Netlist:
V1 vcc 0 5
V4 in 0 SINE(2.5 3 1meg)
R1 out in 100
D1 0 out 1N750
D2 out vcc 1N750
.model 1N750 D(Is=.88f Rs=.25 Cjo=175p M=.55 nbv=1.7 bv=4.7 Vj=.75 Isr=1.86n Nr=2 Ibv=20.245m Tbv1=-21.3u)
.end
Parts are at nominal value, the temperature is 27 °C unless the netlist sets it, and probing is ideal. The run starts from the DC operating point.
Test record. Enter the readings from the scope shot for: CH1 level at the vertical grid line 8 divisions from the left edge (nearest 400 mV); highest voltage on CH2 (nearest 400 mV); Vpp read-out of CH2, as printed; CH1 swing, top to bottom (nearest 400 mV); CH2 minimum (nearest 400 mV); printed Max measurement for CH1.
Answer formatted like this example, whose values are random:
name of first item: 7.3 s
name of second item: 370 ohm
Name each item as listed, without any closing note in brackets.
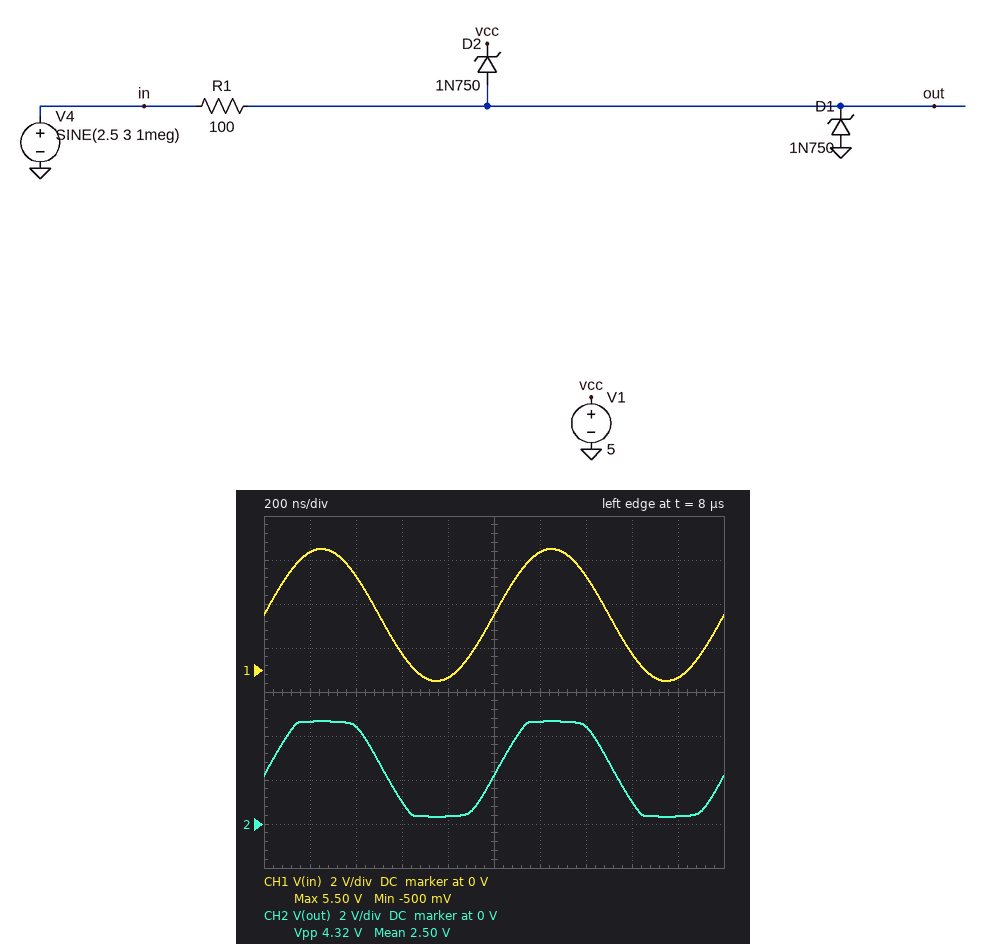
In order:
CH1 level at the vertical grid line 8 divisions from the left edge: 800 mV
highest voltage on CH2: 4.8 V
Vpp read-out of CH2, as printed: 4.32 V
CH1 swing, top to bottom: 6.0 V
CH2 minimum: 400 mV
printed Max measurement for CH1: 5.50 V
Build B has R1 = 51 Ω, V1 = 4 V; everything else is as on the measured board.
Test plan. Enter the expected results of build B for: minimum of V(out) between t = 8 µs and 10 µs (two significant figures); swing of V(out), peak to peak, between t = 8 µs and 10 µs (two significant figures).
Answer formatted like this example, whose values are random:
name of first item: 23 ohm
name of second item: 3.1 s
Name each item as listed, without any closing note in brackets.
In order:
minimum of V(out) between t = 8 µs and 10 µs: -480 mV
swing of V(out), peak to peak, between t = 8 µs and 10 µs: 5.2 V
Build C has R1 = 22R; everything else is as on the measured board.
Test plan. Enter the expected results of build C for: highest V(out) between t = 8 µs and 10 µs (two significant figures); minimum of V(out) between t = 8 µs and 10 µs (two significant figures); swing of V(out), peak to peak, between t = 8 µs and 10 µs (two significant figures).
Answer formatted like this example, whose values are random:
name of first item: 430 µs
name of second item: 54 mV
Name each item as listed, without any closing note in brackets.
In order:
highest V(out) between t = 8 µs and 10 µs: 4.7 V
minimum of V(out) between t = 8 µs and 10 µs: 270 mV
swing of V(out), peak to peak, between t = 8 µs and 10 µs: 4.5 V
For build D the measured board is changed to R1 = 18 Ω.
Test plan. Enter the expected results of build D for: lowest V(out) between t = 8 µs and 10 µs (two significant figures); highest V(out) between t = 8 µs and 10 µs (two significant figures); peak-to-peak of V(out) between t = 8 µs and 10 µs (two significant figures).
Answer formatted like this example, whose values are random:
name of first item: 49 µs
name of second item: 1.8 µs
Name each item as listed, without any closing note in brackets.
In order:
lowest V(out) between t = 8 µs and 10 µs: 260 mV
highest V(out) between t = 8 µs and 10 µs: 4.7 V
peak-to-peak of V(out) between t = 8 µs and 10 µs: 4.5 V
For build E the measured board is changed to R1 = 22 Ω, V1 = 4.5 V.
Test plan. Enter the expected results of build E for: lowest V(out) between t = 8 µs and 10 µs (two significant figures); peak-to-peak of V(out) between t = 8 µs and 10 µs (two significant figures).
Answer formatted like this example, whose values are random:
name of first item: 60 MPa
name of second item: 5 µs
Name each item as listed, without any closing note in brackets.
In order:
lowest V(out) between t = 8 µs and 10 µs: -190 mV
peak-to-peak of V(out) between t = 8 µs and 10 µs: 4.9 V
